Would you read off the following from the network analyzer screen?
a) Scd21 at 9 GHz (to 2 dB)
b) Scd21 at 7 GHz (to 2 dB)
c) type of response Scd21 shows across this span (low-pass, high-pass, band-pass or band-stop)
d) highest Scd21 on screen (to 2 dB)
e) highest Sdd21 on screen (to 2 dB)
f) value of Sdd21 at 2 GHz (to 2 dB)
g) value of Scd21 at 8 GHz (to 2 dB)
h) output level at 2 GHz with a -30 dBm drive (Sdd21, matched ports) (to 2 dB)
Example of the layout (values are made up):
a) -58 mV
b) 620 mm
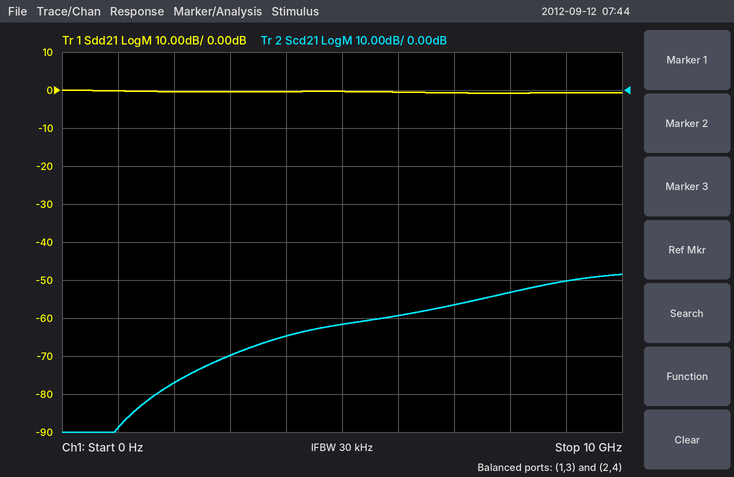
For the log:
a) -50 dB
b) -56 dB
c) high-pass
d) -48 dB
e) 0 dB
f) 0 dB
g) -54 dB
h) -30 dBm
